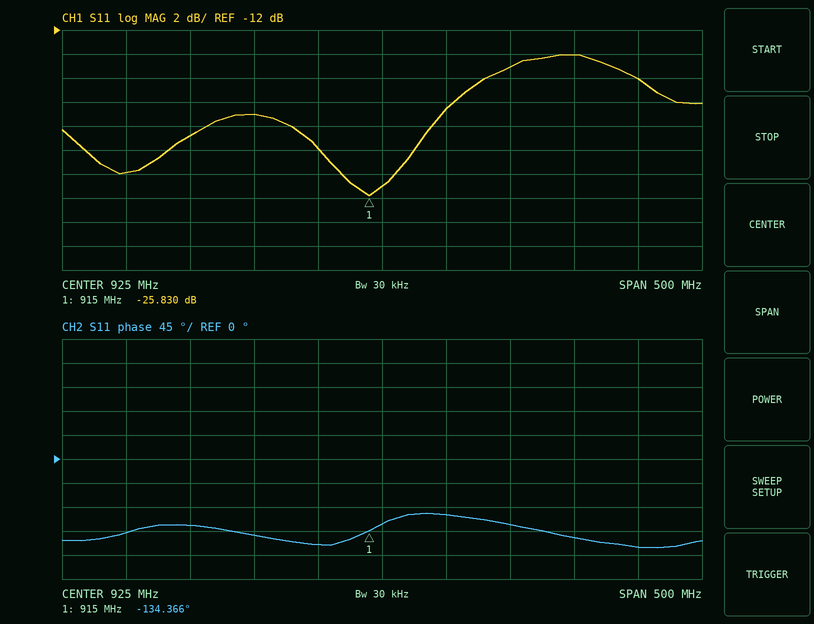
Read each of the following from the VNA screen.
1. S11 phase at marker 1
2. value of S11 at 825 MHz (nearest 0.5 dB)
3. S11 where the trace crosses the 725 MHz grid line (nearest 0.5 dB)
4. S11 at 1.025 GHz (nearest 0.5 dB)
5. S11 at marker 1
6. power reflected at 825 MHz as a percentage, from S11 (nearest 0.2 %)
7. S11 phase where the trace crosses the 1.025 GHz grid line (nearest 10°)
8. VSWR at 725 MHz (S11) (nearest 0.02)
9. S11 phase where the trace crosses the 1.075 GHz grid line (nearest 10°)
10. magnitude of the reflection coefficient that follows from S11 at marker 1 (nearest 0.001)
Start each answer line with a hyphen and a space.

- -134.366°
- -19.0 dB
- -24.0 dB
- -15.0 dB
- -25.830 dB
- 1.2 %
- -120°
- 1.14
- -150°
- 0.051
